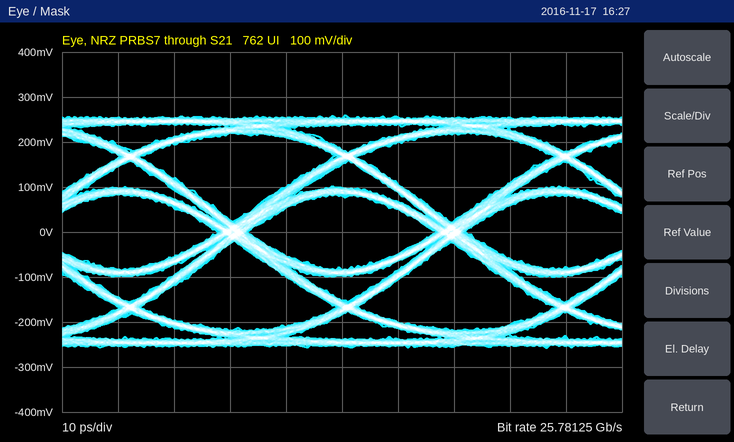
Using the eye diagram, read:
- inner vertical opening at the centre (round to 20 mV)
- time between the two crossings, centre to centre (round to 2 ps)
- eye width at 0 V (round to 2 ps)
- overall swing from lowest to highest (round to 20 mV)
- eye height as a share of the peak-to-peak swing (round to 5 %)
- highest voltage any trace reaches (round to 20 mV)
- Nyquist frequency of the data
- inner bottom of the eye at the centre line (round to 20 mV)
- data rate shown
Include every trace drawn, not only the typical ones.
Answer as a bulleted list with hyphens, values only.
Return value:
- 160 mV
- 38 ps
- 34 ps
- 520 mV
- 30 %
- 260 mV
- 12.89062 GHz
- -80 mV
- 25.78125 Gb/s
